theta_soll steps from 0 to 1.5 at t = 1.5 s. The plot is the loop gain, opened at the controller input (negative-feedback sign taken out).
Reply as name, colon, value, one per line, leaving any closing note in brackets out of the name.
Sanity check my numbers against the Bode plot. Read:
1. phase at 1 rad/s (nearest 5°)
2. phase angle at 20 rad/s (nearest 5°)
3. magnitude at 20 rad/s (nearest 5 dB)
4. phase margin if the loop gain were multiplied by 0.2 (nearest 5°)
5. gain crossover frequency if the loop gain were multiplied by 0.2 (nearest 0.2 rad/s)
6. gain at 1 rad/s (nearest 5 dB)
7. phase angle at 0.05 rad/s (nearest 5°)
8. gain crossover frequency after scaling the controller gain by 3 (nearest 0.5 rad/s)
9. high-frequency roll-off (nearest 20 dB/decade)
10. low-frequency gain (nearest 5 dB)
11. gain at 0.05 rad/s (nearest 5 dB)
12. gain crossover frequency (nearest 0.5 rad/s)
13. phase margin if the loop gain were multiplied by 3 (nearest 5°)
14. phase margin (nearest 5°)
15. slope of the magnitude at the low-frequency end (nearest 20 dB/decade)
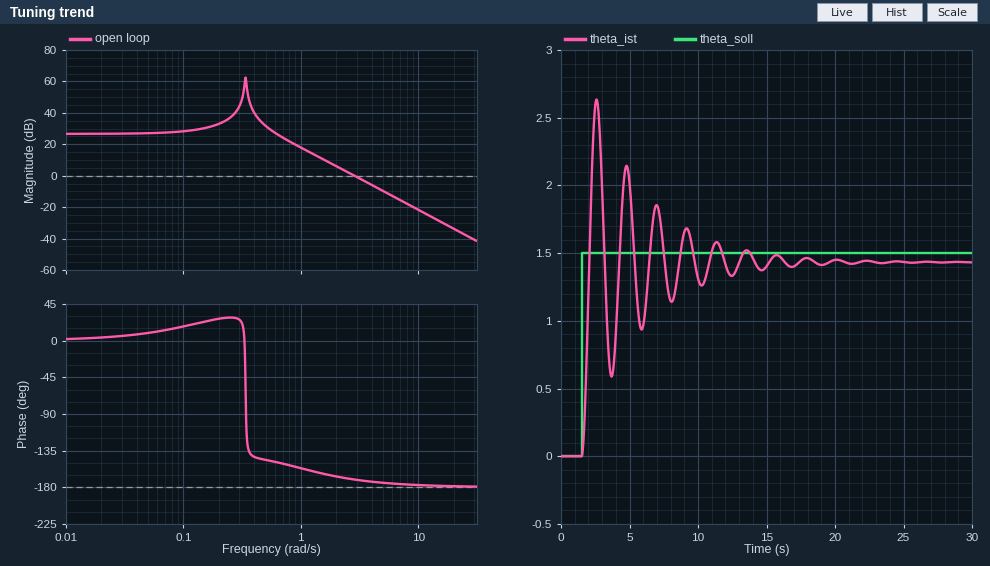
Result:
phase at 1 rad/s: -155°
phase angle at 20 rad/s: -180°
magnitude at 20 rad/s: -35 dB
phase margin if the loop gain were multiplied by 0.2: 20°
gain crossover frequency if the loop gain were multiplied by 0.2: 1.2 rad/s
gain at 1 rad/s: 20 dB
phase angle at 0.05 rad/s: 10°
gain crossover frequency after scaling the controller gain by 3: 5.0 rad/s
high-frequency roll-off: -40 dB/decade
low-frequency gain: 25 dB
gain at 0.05 rad/s: 25 dB
gain crossover frequency: 3.0 rad/s
phase margin if the loop gain were multiplied by 3: 5°
phase margin: 10°
slope of the magnitude at the low-frequency end: 0 dB/decade
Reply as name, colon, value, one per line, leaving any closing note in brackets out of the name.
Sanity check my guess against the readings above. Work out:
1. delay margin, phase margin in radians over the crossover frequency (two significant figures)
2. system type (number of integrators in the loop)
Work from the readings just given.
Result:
delay margin, phase margin in radians over the crossover frequency: 0.058 s
system type: 0
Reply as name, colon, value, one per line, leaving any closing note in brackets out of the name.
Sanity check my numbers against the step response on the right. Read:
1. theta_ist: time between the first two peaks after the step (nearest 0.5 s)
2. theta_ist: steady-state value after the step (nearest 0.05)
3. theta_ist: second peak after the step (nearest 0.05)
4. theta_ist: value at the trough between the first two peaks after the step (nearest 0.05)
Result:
theta_ist: time between the first two peaks after the step: 2.0 s
theta_ist: steady-state value after the step: 1.45
theta_ist: second peak after the step: 2.15
theta_ist: value at the trough between the first two peaks after the step: 0.60
